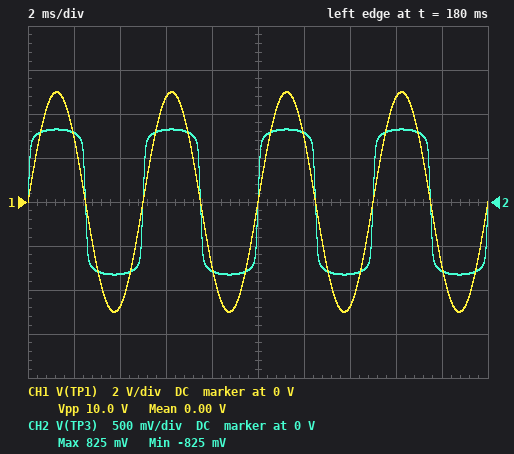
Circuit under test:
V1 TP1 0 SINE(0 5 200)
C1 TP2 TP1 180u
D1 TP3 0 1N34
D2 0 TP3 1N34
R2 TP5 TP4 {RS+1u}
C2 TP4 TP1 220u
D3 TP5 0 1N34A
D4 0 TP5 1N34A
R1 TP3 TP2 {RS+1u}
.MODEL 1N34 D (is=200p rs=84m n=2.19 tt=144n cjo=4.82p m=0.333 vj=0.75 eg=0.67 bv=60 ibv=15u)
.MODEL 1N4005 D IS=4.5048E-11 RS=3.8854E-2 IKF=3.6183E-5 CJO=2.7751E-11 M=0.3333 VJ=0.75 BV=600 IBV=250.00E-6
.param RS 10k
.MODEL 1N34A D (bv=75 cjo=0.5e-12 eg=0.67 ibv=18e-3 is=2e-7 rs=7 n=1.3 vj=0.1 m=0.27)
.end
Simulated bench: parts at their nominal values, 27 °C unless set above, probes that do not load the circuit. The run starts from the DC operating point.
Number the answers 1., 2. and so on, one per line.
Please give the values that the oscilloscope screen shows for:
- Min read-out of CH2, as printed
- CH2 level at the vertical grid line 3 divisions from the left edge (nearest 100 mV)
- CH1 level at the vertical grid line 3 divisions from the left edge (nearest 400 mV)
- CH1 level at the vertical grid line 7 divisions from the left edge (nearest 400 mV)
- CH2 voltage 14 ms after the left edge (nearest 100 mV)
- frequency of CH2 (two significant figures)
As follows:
1. -825 mV
2. 800 mV
3. 4.8 V
4. -4.8 V
5. -800 mV
6. 200 Hz
